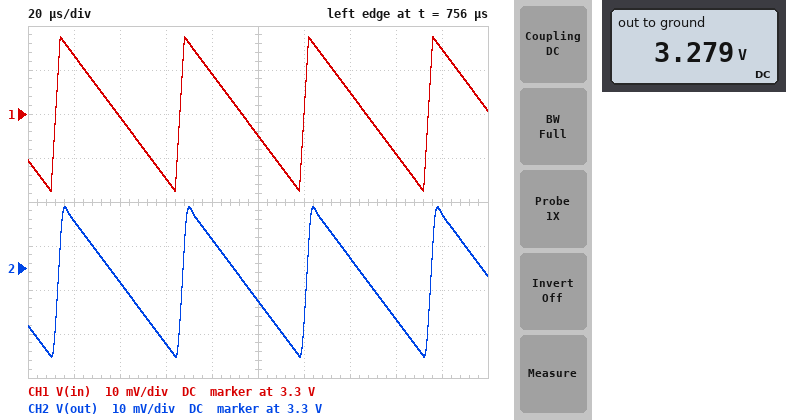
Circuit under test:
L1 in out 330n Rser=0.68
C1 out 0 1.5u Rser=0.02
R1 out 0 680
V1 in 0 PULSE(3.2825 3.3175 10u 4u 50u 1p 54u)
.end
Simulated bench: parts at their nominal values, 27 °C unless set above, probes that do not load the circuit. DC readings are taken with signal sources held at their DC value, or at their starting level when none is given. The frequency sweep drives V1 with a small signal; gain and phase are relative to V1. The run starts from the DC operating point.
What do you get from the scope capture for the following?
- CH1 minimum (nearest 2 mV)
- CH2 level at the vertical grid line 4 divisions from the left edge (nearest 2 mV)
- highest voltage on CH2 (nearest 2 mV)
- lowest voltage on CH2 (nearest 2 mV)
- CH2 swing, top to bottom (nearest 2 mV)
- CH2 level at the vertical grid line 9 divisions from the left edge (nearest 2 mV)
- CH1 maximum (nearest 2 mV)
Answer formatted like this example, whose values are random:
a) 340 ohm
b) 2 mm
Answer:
a) 3.282 V
b) 3.306 V
c) 3.314 V
d) 3.280 V
e) 34 mV
f) 3.312 V
g) 3.318 V
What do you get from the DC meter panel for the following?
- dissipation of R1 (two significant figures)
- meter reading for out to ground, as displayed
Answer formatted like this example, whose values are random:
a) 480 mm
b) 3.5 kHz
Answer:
a) 16 mW
b) 3.279 V
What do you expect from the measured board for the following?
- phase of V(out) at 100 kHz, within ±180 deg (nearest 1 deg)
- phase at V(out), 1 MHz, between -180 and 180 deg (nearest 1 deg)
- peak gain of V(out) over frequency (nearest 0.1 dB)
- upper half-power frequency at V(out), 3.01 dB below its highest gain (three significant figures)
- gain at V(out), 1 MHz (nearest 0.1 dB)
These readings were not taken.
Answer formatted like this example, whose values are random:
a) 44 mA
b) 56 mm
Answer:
a) -38 deg
b) -150 deg
c) 0 dB
d) 214 kHz
e) -25.7 dB
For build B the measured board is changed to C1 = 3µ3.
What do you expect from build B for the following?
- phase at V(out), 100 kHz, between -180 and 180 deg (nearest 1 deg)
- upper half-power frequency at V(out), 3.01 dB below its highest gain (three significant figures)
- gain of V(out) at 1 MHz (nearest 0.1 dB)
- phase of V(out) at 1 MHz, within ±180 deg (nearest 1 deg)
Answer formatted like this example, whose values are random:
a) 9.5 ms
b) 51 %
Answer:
a) -66 deg
b) 85.3 kHz
c) -32.3 dB
d) -138 deg
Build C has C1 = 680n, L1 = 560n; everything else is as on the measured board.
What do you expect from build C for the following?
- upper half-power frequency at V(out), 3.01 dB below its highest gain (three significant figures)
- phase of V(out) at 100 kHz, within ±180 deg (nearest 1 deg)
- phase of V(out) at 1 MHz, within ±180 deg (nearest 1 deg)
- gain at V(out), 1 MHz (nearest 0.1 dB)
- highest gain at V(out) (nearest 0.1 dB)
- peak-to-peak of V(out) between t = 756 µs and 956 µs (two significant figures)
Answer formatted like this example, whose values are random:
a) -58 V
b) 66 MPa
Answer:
a) 307 kHz
b) -19 deg
c) -163 deg
d) -23.1 dB
e) 2.9 dB
f) 37 mV
